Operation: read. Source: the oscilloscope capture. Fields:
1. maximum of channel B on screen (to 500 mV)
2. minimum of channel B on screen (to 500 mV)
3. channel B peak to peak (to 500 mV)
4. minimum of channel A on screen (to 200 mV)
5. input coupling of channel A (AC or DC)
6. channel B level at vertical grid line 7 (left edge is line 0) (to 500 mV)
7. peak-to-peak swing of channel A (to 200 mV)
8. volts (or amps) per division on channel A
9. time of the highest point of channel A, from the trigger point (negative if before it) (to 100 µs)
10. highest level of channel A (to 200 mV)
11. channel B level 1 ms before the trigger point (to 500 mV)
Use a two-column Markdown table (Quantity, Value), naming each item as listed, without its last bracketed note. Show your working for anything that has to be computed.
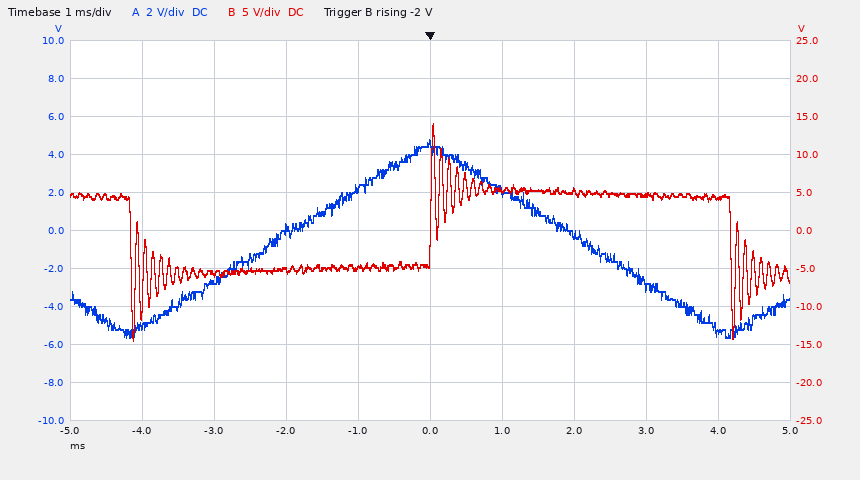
| Quantity | Value |
|---|---|
| maximum of channel B on screen | 14.0 V |
| minimum of channel B on screen | -14.5 V |
| channel B peak to peak | 14.0 V − (-14.5 V) = 28.5 V |
| minimum of channel A on screen | -5.6 V |
| input coupling of channel A | DC |
| channel B level at vertical grid line 7 (left edge is line 0) | 5.0 V |
| peak-to-peak swing of channel A | 4.8 V − (-5.6 V) = 10.4 V |
| volts (or amps) per division on channel A | 2 V |
| time of the highest point of channel A, from the trigger point (negative if before it) | 0.0 ms |
| highest level of channel A | 4.8 V |
| channel B level 1 ms before the trigger point | -5.0 V |
